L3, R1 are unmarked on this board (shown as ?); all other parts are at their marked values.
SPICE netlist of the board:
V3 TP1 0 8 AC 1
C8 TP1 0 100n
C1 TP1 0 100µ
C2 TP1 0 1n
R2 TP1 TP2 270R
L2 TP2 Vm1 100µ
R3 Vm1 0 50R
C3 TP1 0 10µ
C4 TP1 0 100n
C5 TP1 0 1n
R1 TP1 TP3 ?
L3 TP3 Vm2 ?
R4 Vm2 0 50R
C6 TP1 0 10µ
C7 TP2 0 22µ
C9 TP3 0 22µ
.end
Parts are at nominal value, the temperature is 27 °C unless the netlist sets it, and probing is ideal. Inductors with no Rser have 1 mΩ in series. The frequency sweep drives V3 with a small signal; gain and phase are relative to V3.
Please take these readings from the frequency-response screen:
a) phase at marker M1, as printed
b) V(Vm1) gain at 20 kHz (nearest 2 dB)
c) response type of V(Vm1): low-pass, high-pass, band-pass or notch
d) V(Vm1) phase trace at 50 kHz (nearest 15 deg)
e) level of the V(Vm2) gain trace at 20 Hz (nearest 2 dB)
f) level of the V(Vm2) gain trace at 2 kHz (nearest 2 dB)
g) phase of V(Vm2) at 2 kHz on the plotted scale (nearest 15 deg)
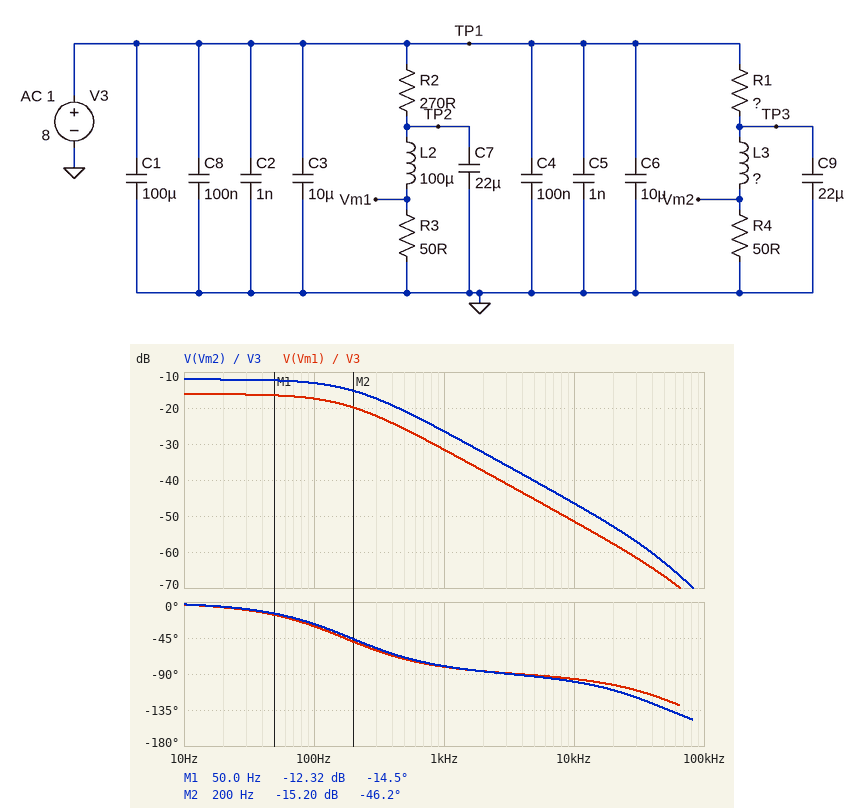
-14.5 deg
-58 dB
low-pass
-120 deg
-12 dB
-32 dB
-90 deg
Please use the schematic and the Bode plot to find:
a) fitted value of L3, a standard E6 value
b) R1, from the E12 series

150 µH
150 Ω
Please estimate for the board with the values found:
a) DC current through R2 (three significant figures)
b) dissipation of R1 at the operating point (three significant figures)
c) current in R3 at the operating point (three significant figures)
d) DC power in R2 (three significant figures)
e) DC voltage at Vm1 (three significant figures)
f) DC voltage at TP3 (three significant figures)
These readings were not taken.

25.0 mA
240 mW
25.0 mA
169 mW
1.25 V
2.00 V
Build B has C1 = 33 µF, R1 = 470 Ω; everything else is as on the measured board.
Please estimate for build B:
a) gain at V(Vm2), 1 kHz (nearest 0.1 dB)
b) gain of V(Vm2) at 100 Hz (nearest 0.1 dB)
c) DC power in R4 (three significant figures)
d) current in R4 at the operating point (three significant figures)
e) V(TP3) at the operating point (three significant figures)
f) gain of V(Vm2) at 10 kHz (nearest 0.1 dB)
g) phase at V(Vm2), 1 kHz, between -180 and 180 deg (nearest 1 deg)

-36.3 dB
-21.8 dB
11.8 mW
15.4 mA
769 mV
-56.4 dB
-82 deg
